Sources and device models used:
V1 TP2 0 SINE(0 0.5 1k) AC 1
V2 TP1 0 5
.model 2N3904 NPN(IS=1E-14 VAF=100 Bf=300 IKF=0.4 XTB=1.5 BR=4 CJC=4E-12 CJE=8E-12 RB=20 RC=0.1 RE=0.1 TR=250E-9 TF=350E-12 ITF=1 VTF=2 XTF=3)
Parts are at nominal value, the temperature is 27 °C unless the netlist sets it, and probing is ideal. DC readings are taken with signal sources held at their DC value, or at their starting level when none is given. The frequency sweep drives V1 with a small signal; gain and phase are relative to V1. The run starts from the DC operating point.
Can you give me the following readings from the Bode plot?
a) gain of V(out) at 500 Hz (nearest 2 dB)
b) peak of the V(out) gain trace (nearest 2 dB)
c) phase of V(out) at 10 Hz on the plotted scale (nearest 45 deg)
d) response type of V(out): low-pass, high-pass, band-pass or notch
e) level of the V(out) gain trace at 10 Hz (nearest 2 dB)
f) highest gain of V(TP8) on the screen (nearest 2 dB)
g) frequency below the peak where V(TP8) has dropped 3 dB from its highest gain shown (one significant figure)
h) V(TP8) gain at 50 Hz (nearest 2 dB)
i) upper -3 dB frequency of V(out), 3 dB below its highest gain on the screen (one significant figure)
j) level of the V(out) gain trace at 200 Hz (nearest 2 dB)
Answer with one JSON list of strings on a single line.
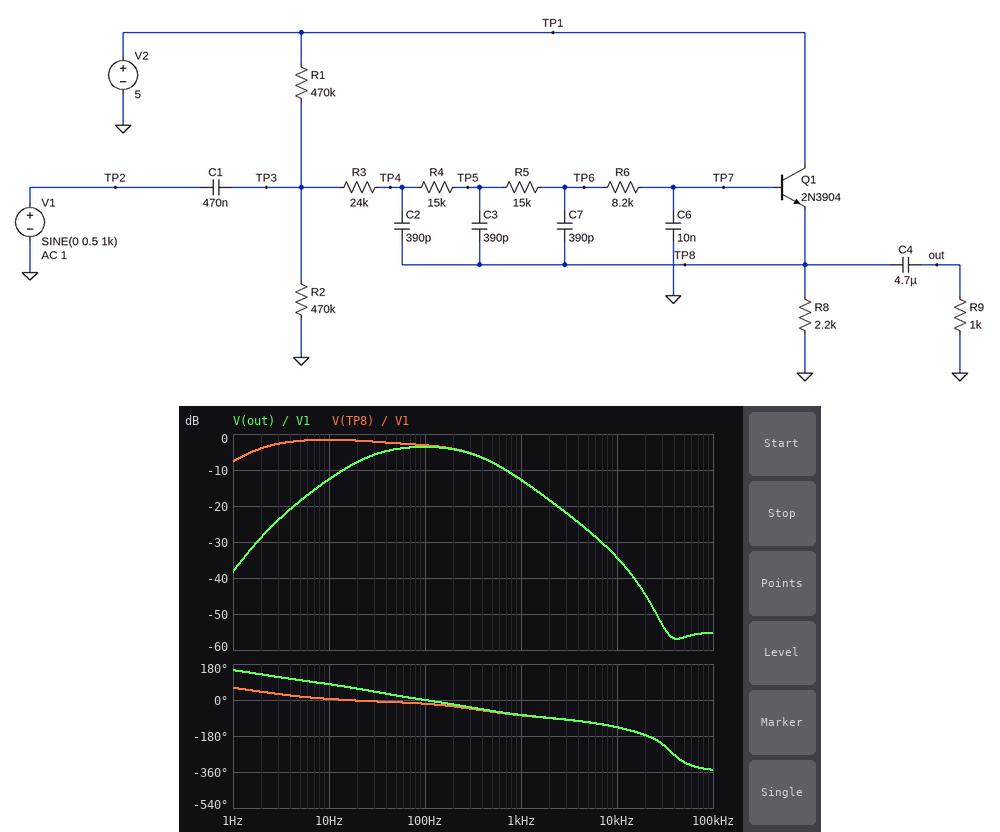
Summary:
["-8 dB", "-4 dB", "90 deg", "band-pass", "-12 dB", "-2 dB", "2 Hz", "-2 dB", "400 Hz", "-4 dB"]
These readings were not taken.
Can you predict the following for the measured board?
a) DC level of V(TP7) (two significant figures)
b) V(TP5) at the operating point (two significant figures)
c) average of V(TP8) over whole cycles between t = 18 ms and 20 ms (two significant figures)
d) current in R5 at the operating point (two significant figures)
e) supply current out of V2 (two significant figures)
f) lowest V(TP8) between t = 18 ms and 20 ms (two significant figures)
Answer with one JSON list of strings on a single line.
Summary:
["1.9 V", "2.0 V", "1.3 V", "1.9 µA", "590 µA", "1.2 V"]
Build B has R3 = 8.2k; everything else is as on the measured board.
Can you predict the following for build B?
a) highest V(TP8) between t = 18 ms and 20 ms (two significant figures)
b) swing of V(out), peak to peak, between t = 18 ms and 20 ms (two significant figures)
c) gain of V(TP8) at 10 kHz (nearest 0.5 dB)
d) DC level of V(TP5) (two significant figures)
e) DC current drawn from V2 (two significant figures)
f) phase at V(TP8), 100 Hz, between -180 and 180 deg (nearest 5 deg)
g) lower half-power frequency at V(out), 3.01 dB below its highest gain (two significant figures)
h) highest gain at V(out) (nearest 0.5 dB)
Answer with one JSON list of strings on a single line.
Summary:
["1.5 V", "300 mV", "-31.0 dB", "2.0 V", "600 µA", "-15 deg", "26 Hz", "-3.0 dB"]
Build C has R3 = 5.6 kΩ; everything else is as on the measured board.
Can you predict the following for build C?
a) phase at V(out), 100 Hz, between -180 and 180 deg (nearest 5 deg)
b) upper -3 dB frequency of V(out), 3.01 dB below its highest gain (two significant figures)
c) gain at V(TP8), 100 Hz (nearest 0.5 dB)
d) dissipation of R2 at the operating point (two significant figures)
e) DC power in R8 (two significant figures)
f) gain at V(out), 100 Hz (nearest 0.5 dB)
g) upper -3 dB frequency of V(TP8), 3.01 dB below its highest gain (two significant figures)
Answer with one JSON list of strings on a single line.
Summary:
["5 deg", "510 Hz", "-2.5 dB", "8.9 µW", "790 µW", "-3.0 dB", "360 Hz"]
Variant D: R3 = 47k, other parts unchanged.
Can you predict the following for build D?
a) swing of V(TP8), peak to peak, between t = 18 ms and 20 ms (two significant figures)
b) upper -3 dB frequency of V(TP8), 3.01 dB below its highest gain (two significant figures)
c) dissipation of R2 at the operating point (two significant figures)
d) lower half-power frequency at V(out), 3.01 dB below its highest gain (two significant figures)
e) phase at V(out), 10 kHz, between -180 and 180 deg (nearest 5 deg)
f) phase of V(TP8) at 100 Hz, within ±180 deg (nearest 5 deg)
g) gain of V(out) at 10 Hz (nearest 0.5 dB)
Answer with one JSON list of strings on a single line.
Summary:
["170 mV", "160 Hz", "9.1 µW", "23 Hz", "-145 deg", "-25 deg", "-13.0 dB"]
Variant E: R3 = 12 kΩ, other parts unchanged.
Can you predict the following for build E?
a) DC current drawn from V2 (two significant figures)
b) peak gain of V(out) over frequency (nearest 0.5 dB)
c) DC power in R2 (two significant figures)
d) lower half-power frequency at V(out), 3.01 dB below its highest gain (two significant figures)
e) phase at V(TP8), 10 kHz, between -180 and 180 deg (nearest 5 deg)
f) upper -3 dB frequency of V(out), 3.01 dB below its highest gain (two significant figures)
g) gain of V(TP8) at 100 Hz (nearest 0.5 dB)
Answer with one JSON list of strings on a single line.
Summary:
["600 µA", "-3.0 dB", "8.9 µW", "26 Hz", "-125 deg", "460 Hz", "-2.5 dB"]
